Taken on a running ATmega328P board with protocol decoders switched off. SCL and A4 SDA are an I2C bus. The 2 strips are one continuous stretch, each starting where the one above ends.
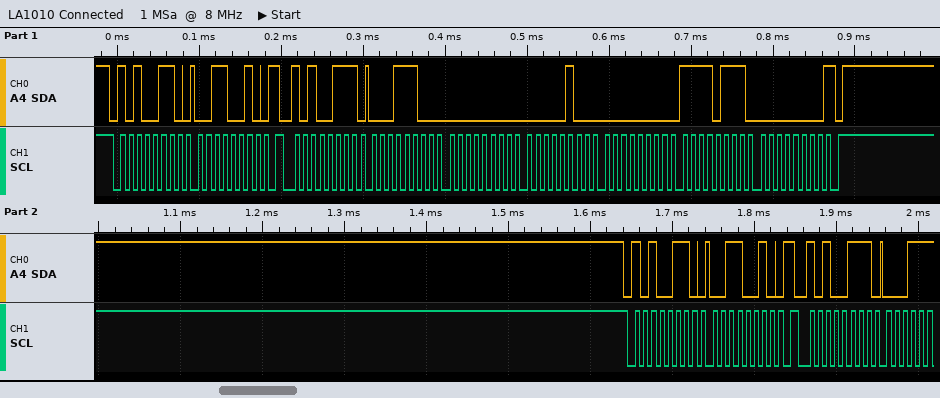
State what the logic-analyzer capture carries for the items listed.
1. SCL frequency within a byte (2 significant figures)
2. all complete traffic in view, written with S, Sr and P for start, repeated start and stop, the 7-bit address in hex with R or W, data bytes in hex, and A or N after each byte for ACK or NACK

100 kHz
S 53W A 32 A Sr 53R A 1C A 00 A 04 A 00 A F7 A 00 N P S 53W A 32 A Sr 53R A
